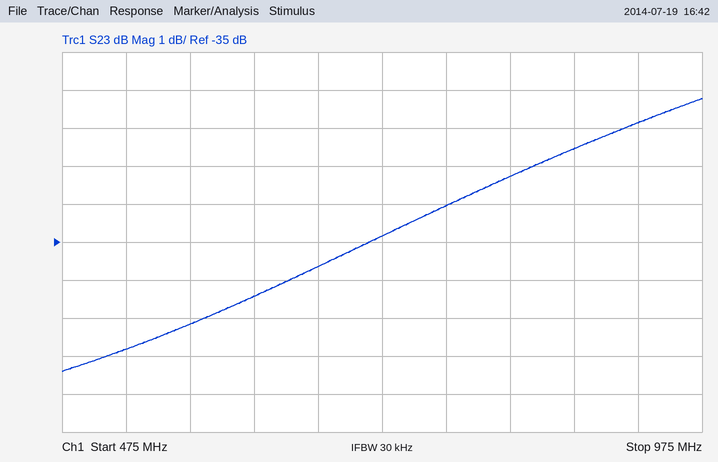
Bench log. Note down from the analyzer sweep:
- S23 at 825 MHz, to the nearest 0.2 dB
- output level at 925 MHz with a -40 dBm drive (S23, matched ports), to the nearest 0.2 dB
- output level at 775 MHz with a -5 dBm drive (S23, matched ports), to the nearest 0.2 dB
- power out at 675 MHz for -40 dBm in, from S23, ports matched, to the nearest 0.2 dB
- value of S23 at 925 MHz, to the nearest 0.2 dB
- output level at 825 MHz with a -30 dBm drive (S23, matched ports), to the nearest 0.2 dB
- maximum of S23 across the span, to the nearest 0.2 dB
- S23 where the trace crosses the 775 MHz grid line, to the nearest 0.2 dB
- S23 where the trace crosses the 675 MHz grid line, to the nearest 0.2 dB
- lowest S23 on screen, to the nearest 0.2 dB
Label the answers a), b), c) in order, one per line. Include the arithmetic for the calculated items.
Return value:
a) -33.2 dB
b) -40 dBm + (-31.8 dB) = -71.8 dBm
c) -5 dBm + (-34.0 dB) = -39.0 dBm
d) -40 dBm + (-35.6 dB) = -75.6 dBm
e) -31.8 dB
f) -30 dBm + (-33.2 dB) = -63.2 dBm
g) -31.2 dB
h) -34.0 dB
i) -35.6 dB
j) -38.4 dB
